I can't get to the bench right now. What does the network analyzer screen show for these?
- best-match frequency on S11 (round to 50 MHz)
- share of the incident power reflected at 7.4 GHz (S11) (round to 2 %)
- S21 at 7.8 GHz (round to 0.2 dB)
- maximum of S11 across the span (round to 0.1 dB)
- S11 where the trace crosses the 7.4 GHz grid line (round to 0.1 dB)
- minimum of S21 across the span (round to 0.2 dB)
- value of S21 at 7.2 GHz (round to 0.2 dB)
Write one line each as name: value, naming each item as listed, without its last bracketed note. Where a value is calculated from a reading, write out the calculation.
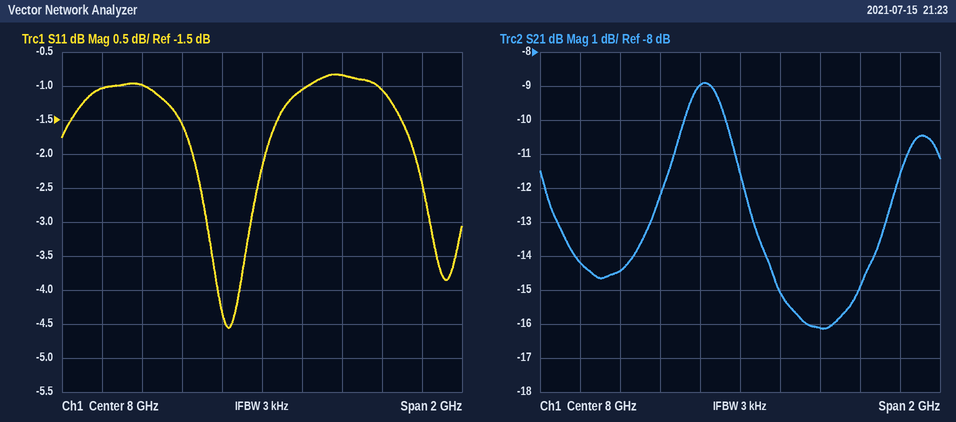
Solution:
best-match frequency on S11: 7.85 GHz
share of the incident power reflected at 7.4 GHz (S11): 10^(-1/10) ≈ 79.4 %, so 80 % to the nearest 2 %
S21 at 7.8 GHz: -9.0 dB
maximum of S11 across the span: -0.8 dB
S11 where the trace crosses the 7.4 GHz grid line: -1.0 dB
minimum of S21 across the span: -16.2 dB
value of S21 at 7.2 GHz: -14.2 dB
